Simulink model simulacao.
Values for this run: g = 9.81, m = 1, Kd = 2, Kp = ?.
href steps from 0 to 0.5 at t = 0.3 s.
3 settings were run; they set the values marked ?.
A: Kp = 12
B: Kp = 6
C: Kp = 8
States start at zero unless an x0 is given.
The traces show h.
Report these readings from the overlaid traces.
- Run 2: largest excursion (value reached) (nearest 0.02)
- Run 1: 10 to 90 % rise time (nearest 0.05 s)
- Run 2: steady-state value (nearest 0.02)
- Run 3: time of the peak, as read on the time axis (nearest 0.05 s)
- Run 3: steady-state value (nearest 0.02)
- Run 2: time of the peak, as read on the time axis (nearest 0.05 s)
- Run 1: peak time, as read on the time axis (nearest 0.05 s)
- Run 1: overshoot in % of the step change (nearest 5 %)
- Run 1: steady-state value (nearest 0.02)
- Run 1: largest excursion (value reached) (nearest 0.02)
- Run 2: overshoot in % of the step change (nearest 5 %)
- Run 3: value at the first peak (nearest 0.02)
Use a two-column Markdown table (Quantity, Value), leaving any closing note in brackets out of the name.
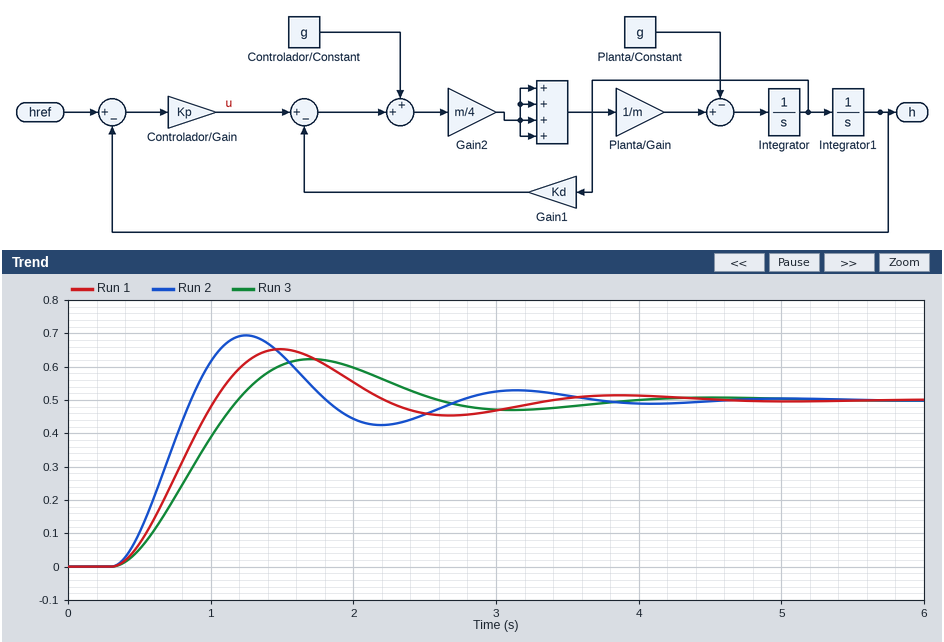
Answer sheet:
| Quantity | Value |
|---|---|
| Run 2: largest excursion (value reached) | 0.70 |
| Run 1: 10 to 90 % rise time | 0.50 s |
| Run 2: steady-state value | 0.50 |
| Run 3: time of the peak, as read on the time axis | 1.70 s |
| Run 3: steady-state value | 0.50 |
| Run 2: time of the peak, as read on the time axis | 1.25 s |
| Run 1: peak time, as read on the time axis | 1.50 s |
| Run 1: overshoot in % of the step change | 30 % |
| Run 1: steady-state value | 0.50 |
| Run 1: largest excursion (value reached) | 0.66 |
| Run 2: overshoot in % of the step change | 40 % |
| Run 3: value at the first peak | 0.62 |
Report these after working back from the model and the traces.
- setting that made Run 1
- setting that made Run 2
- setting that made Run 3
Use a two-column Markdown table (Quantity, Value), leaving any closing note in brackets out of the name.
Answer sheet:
| Quantity | Value |
|---|---|
| setting that made Run 1 | C |
| setting that made Run 2 | A |
| setting that made Run 3 | B |
